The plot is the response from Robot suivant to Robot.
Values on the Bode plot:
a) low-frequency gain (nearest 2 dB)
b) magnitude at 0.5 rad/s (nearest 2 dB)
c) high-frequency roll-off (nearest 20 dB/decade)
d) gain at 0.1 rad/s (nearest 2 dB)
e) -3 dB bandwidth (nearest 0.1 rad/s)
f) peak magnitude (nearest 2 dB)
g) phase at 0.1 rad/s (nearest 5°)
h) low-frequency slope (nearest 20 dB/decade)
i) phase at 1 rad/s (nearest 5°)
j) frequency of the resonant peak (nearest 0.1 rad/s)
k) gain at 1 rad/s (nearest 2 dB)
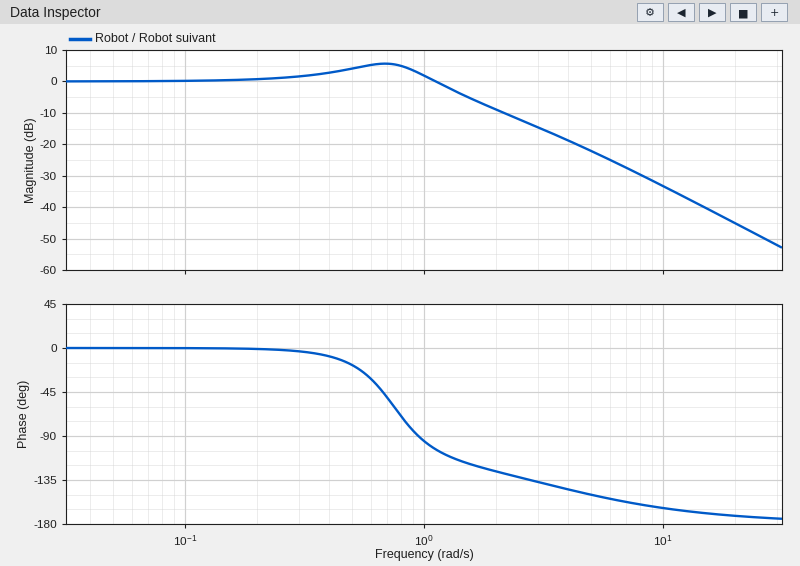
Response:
0 dB
4 dB
-40 dB/decade
0 dB
1.3 rad/s
6 dB
0°
0 dB/decade
-95°
0.7 rad/s
2 dB
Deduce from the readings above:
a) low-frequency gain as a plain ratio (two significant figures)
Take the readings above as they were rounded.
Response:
1.0
